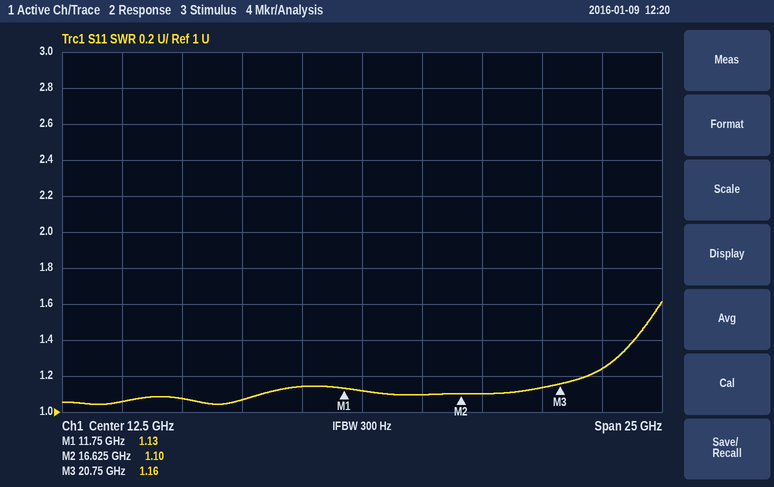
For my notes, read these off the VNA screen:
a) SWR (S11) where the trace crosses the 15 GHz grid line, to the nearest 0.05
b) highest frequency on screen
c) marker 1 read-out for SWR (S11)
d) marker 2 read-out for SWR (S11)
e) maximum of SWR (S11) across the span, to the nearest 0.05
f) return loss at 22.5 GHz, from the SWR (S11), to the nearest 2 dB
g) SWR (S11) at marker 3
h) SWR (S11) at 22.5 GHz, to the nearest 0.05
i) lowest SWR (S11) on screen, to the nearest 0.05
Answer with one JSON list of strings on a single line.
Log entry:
["1.10", "25 GHz", "1.13", "1.10", "1.60", "20 dB", "1.16", "1.25", "1.05"]
